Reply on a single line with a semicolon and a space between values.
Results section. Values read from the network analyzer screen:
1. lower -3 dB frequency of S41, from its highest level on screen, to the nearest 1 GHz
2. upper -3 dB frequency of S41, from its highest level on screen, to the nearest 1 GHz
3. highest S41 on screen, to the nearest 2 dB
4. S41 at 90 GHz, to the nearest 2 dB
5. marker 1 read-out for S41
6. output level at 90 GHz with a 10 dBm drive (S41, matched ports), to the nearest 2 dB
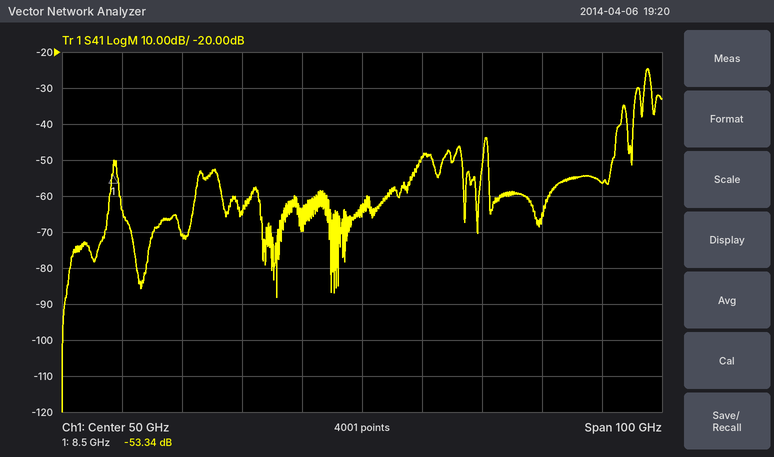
97 GHz; 98 GHz; -24 dB; -56 dB; -53.34 dB; -46 dBm
